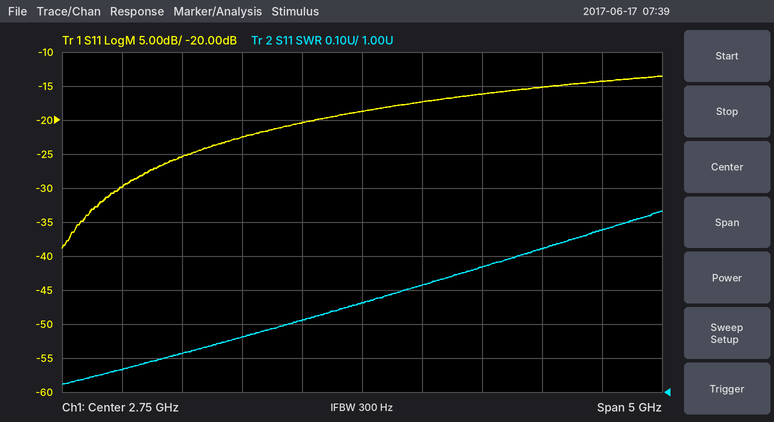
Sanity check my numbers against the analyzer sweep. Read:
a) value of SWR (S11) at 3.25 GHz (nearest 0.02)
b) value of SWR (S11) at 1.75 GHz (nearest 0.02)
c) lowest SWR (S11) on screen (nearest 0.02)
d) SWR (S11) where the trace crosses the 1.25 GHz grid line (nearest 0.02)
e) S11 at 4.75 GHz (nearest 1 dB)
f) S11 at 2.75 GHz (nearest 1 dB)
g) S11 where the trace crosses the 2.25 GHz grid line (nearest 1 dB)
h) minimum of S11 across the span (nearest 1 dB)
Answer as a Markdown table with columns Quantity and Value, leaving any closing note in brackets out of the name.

| Quantity | Value |
|---|---|
| value of SWR (S11) at 3.25 GHz | 1.32 |
| value of SWR (S11) at 1.75 GHz | 1.16 |
| lowest SWR (S11) on screen | 1.02 |
| SWR (S11) where the trace crosses the 1.25 GHz grid line | 1.12 |
| S11 at 4.75 GHz | -14 dB |
| S11 at 2.75 GHz | -19 dB |
| S11 where the trace crosses the 2.25 GHz grid line | -20 dB |
| minimum of S11 across the span | -39 dB |
